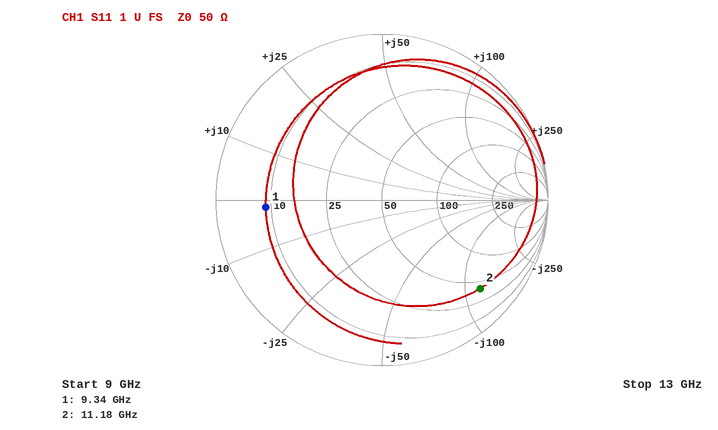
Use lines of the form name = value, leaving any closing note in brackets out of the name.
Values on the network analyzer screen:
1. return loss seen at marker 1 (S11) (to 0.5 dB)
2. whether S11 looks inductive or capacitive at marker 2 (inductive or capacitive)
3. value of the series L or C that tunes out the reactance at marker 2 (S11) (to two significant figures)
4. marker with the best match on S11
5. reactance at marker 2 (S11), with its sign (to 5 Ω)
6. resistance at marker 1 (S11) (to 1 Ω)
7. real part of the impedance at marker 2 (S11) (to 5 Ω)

return loss seen at marker 1 (S11) = 3.0 dB
whether S11 looks inductive or capacitive at marker 2 = capacitive
value of the series L or C that tunes out the reactance at marker 2 (S11) = 1.7 nH
marker with the best match on S11 = marker 1
reactance at marker 2 (S11), with its sign = -120 Ω
resistance at marker 1 (S11) = 9 Ω
real part of the impedance at marker 2 (S11) = 40 Ω
